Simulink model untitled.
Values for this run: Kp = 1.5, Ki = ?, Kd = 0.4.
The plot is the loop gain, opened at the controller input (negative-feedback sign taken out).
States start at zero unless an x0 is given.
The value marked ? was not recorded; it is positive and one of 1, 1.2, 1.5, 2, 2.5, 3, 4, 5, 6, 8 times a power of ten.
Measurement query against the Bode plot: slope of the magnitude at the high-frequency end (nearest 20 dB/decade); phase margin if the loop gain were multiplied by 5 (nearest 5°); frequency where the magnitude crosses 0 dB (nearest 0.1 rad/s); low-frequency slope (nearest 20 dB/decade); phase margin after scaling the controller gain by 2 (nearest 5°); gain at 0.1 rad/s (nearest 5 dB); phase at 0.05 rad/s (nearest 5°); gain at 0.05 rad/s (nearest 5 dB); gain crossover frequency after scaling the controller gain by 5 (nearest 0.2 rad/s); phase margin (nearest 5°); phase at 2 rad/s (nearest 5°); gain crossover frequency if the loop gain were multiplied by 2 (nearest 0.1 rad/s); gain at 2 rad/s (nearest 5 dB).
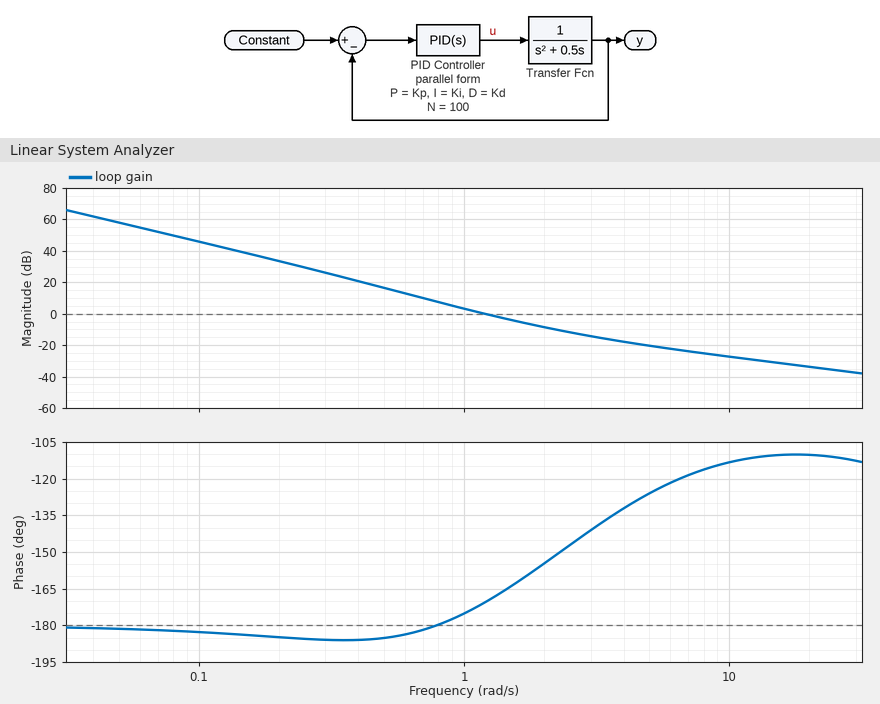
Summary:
-20 dB/decade
40°
1.2 rad/s
-40 dB/decade
20°
45 dB
-180°
60 dB
3.0 rad/s
10°
-155°
1.7 rad/s
-10 dB
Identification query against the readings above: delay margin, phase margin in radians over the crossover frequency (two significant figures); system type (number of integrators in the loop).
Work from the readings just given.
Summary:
0.15 s
2
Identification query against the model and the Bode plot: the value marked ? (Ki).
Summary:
1
